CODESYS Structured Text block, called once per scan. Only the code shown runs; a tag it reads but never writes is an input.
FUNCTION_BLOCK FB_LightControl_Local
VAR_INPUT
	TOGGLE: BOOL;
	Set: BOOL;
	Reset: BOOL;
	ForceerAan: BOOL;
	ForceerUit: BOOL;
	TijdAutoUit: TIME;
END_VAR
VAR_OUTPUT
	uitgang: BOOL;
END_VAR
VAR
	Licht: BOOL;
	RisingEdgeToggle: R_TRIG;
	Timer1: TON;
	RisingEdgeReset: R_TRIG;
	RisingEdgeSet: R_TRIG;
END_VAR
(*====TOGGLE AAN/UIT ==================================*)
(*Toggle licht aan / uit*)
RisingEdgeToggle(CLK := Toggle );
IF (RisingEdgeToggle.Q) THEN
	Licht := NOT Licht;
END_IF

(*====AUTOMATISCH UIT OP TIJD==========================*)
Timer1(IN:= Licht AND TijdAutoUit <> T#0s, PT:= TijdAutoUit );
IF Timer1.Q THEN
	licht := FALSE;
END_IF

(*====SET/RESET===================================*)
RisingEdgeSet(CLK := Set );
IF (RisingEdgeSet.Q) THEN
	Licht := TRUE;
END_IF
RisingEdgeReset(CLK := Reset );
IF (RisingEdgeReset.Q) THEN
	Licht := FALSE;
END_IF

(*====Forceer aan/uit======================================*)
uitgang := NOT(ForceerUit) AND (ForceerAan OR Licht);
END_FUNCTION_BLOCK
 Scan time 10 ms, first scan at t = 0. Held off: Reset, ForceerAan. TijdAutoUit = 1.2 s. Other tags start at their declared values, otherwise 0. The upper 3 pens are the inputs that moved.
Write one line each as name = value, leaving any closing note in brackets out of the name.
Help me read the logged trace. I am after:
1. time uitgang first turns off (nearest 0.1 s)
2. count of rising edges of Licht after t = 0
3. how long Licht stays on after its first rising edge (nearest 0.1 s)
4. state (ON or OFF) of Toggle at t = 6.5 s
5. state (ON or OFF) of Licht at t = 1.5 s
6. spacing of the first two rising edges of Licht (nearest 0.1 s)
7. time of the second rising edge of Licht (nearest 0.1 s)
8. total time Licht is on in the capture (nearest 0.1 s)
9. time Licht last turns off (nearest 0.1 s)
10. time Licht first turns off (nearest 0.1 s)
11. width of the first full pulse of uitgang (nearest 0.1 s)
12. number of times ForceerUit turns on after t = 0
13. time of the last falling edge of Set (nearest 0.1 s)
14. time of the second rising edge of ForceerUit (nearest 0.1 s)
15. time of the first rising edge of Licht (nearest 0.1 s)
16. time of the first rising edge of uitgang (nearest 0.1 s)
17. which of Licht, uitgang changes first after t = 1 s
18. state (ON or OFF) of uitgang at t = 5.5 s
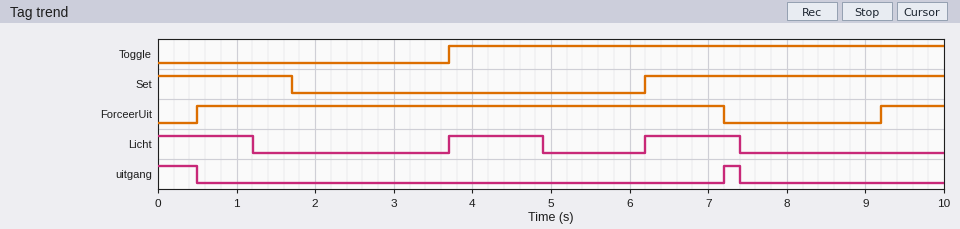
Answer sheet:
time uitgang first turns off = 0.5 s
count of rising edges of Licht after t = 0 = 2
how long Licht stays on after its first rising edge = 1.2 s
state (ON or OFF) of Toggle at t = 6.5 s = ON
state (ON or OFF) of Licht at t = 1.5 s = OFF
spacing of the first two rising edges of Licht = 2.5 s
time of the second rising edge of Licht = 6.2 s
total time Licht is on in the capture = 3.6 s
time Licht last turns off = 7.4 s
time Licht first turns off = 1.2 s
width of the first full pulse of uitgang = 0.2 s
number of times ForceerUit turns on after t = 0 = 2
time of the last falling edge of Set = 1.7 s
time of the second rising edge of ForceerUit = 9.2 s
time of the first rising edge of Licht = 3.7 s
time of the first rising edge of uitgang = 7.2 s
which of Licht, uitgang changes first after t = 1 s = Licht
state (ON or OFF) of uitgang at t = 5.5 s = OFF
